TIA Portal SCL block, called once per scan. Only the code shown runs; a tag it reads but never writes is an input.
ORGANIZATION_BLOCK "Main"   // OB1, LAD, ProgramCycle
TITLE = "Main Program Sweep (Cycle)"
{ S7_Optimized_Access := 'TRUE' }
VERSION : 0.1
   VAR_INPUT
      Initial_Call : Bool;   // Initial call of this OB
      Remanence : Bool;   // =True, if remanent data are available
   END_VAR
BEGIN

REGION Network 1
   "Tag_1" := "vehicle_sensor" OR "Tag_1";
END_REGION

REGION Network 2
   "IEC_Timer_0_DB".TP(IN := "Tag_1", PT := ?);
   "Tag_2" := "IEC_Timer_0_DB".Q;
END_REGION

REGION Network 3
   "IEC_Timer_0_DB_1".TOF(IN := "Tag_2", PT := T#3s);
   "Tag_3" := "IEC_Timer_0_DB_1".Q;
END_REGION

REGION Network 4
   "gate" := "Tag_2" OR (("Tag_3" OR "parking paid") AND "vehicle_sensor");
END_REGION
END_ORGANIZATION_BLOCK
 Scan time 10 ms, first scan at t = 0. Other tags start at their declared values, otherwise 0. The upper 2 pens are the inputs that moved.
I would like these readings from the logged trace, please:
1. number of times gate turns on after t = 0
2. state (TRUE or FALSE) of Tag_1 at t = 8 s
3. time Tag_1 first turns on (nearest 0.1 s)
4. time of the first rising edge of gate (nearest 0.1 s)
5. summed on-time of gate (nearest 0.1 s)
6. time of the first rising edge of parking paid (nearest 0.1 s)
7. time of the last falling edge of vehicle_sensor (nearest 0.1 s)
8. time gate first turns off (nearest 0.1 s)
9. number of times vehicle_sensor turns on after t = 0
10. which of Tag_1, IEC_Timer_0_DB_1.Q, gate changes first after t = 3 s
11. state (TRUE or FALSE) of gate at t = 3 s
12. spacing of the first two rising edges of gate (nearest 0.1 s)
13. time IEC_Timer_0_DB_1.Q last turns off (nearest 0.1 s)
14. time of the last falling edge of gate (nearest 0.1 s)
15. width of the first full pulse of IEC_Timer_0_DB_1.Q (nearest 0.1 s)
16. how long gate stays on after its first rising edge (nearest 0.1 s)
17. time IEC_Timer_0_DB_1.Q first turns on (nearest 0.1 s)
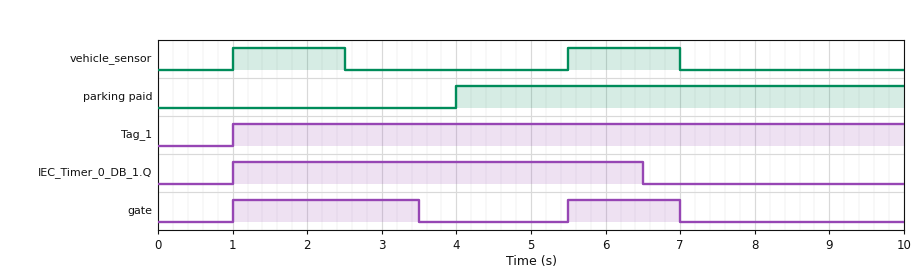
2
TRUE
1.0 s
1.0 s
4.0 s
4.0 s
7.0 s
3.5 s
2
gate
TRUE
4.5 s
6.5 s
7.0 s
5.5 s
2.5 s
1.0 s
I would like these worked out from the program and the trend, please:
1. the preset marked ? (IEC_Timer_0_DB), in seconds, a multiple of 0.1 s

2.5 s
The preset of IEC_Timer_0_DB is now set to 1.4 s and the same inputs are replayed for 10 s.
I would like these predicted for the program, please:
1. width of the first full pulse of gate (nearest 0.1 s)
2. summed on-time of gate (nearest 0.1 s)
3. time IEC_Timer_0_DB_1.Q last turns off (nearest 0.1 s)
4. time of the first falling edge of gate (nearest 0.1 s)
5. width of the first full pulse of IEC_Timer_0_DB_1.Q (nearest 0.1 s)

1.5 s
3.0 s
5.4 s
2.5 s
4.4 s
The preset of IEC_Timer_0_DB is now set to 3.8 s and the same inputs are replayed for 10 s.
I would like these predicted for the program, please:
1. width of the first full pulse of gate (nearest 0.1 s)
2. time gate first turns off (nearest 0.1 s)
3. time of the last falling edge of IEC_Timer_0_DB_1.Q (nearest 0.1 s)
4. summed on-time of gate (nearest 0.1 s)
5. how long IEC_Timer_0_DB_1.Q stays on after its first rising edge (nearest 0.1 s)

3.8 s
4.8 s
7.8 s
5.3 s
6.8 s
